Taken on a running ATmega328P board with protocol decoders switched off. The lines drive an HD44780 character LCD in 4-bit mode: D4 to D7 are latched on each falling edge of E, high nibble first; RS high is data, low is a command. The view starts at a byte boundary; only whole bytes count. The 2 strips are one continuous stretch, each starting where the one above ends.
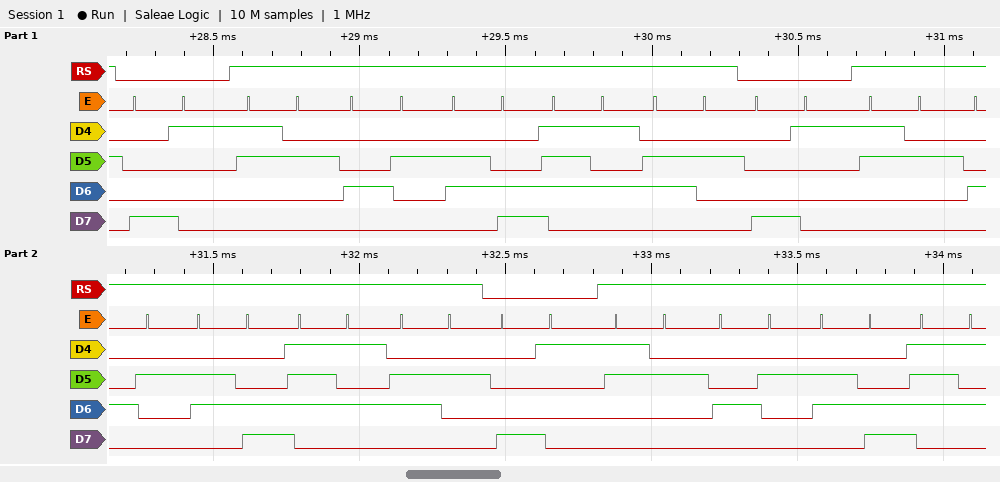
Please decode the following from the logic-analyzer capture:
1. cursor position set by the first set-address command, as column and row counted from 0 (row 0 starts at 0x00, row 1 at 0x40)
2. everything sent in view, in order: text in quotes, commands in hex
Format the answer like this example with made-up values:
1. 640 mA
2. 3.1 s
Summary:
1. column 1, row 0
2. 0x81 "2Blub" 0x81 "2Blub" 0x81 "2Blu"
